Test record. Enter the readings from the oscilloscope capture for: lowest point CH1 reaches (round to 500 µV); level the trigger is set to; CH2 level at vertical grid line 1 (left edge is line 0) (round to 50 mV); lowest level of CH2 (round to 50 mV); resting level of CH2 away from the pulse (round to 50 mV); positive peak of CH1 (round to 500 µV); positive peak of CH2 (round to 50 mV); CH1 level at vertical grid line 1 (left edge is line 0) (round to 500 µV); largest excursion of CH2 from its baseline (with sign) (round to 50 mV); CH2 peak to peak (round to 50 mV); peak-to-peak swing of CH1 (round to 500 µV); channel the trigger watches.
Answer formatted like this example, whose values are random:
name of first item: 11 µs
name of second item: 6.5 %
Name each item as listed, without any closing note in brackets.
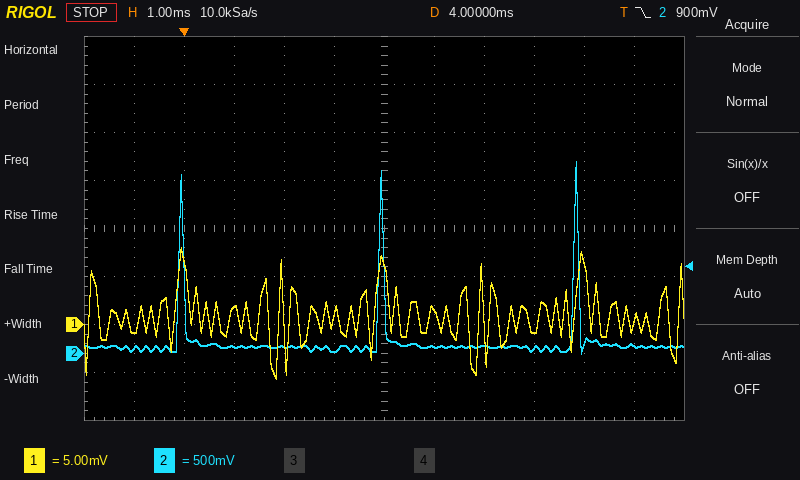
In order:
lowest point CH1 reaches: -5.5 mV
level the trigger is set to: 900 mV
CH2 level at vertical grid line 1 (left edge is line 0): 50 mV
lowest level of CH2: 0 mV
resting level of CH2 away from the pulse: 50 mV
positive peak of CH1: 8.0 mV
positive peak of CH2: 2.00 V
CH1 level at vertical grid line 1 (left edge is line 0): -500 µV
largest excursion of CH2 from its baseline (with sign): +1.95 V
CH2 peak to peak: 2.00 V
peak-to-peak swing of CH1: 13.5 mV
channel the trigger watches: CH2
